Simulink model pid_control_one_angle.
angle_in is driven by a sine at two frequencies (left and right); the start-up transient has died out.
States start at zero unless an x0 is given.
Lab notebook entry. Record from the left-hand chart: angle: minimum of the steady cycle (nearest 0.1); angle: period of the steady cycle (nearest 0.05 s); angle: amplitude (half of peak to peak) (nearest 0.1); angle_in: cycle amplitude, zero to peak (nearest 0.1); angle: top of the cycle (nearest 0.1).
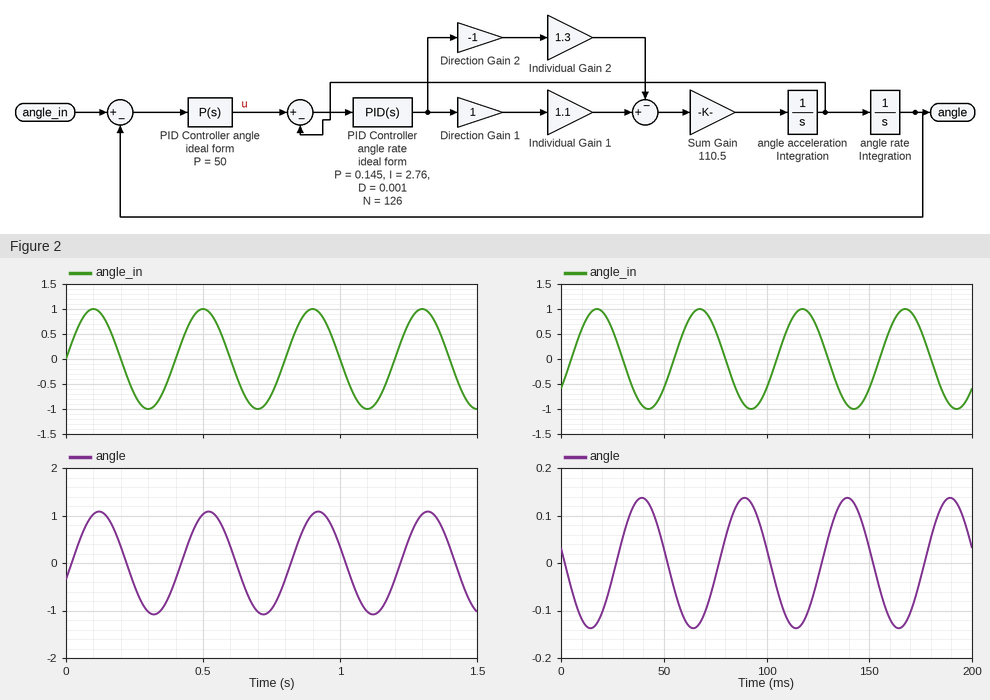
-1.1
0.40 s
1.1
1.0
1.1
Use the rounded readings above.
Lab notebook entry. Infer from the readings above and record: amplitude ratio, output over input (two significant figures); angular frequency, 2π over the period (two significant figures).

1.1
16 rad/s
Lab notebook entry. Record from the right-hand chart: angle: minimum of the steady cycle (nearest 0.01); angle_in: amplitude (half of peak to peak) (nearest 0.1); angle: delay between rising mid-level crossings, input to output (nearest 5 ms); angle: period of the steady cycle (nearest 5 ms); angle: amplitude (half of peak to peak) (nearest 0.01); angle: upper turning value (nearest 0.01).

-0.14
1.0
20 ms
50 ms
0.14
0.14
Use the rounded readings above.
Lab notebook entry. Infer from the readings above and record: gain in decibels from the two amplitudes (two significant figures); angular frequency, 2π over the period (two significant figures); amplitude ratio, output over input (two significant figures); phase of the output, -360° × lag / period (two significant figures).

-17 dB
0.13 rad/ms
0.14
-140°
